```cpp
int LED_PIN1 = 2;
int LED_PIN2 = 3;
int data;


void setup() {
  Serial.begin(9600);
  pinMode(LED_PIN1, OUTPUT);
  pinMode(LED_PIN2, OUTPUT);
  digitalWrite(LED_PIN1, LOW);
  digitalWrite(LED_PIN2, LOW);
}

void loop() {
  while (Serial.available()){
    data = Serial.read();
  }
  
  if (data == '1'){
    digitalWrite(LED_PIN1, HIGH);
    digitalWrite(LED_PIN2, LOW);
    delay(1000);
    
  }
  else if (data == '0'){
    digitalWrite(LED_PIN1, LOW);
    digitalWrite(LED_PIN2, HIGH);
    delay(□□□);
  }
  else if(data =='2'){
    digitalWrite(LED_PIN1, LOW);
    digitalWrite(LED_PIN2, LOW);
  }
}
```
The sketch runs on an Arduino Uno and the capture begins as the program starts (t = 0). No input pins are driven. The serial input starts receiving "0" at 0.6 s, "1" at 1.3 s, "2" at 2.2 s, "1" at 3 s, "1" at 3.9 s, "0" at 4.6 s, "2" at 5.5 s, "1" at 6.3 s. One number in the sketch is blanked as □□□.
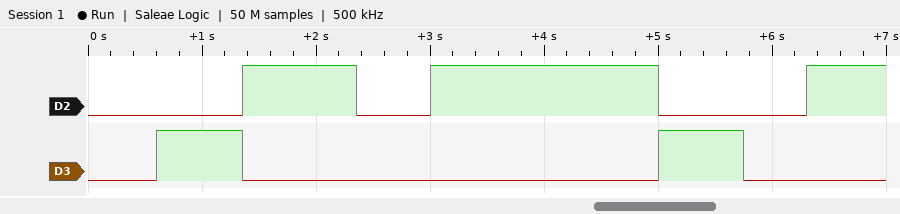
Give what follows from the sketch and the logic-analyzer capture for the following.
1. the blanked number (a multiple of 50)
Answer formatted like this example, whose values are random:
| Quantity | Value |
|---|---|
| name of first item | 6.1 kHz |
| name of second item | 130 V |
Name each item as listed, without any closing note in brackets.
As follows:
| Quantity | Value |
|---|---|
| the blanked number | 750 |
